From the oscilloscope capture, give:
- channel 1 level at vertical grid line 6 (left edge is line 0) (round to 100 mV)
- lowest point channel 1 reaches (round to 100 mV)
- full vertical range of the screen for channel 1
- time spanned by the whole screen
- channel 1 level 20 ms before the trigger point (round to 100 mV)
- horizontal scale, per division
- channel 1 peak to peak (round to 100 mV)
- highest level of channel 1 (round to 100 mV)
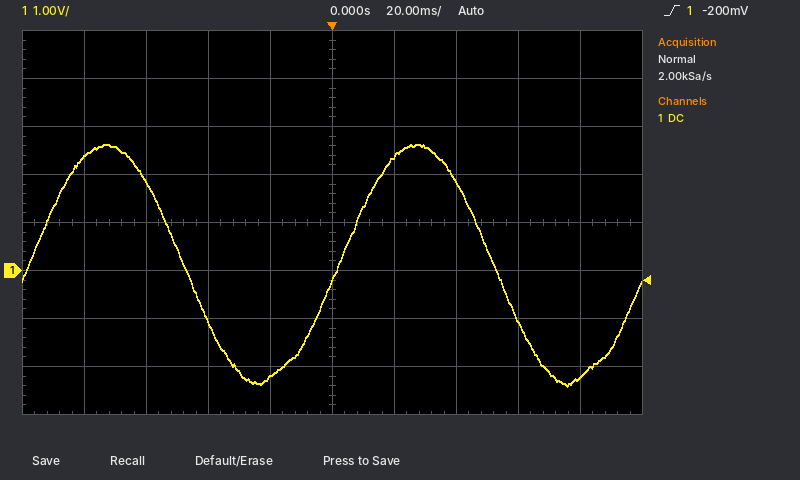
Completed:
2.4 V
-2.4 V
8 V
200 ms
-2.2 V
20 ms
5.0 V
2.6 V
